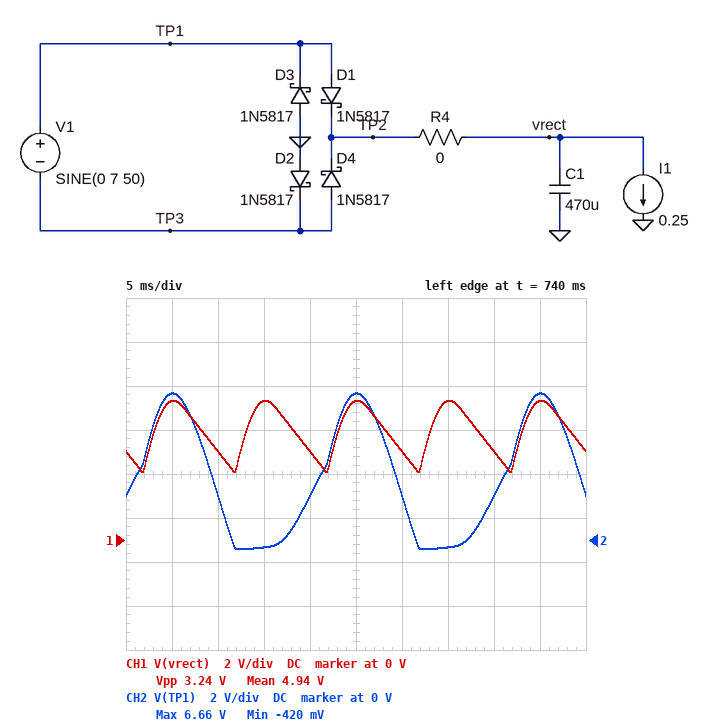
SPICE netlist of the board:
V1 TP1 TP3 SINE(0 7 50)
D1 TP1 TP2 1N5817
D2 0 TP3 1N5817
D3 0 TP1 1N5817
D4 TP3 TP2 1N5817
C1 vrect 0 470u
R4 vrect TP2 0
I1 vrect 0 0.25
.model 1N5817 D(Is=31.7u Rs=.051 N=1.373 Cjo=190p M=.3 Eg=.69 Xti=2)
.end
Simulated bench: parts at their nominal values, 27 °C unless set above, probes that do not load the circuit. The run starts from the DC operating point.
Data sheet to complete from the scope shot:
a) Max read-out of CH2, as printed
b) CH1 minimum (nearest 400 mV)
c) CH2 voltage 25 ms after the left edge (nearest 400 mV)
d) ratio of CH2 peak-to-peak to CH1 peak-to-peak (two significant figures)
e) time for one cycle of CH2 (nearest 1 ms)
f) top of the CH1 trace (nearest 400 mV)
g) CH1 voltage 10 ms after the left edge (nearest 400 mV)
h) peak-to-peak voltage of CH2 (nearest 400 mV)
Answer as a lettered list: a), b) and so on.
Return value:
a) 6.66 V
b) 3.2 V
c) 6.8 V
d) 2.2
e) 20 ms
f) 6.4 V
g) 4.0 V
h) 7.2 V
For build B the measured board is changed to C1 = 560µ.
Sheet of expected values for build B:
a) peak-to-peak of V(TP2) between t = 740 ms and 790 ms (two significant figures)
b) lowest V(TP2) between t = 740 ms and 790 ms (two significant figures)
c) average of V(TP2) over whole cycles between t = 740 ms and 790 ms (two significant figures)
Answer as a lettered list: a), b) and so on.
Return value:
a) 2.8 V
b) 3.5 V
c) 5.1 V
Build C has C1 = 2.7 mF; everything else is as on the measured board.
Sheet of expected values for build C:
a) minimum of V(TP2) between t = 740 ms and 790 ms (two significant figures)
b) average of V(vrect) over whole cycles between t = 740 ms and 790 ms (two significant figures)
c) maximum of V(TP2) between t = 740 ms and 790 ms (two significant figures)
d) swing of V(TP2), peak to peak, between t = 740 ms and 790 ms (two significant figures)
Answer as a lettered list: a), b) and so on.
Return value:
a) 5.5 V
b) 5.9 V
c) 6.2 V
d) 710 mV
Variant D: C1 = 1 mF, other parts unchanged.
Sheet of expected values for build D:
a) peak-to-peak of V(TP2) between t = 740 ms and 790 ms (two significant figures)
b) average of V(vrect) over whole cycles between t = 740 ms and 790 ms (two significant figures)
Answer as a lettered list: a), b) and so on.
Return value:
a) 1.8 V
b) 5.5 V
